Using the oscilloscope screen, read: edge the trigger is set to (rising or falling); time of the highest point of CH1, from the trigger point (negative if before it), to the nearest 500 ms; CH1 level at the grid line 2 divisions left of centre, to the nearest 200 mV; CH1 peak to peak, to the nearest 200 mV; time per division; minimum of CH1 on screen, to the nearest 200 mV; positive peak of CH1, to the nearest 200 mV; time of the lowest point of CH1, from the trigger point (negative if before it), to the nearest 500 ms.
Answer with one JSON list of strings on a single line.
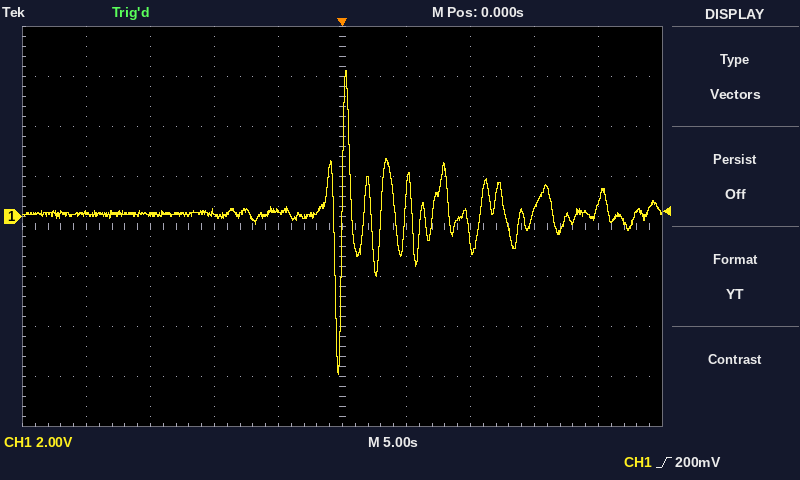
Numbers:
["rising", "+500 ms", "200 mV", "12.2 V", "5 s", "-6.4 V", "5.8 V", "-500 ms"]
